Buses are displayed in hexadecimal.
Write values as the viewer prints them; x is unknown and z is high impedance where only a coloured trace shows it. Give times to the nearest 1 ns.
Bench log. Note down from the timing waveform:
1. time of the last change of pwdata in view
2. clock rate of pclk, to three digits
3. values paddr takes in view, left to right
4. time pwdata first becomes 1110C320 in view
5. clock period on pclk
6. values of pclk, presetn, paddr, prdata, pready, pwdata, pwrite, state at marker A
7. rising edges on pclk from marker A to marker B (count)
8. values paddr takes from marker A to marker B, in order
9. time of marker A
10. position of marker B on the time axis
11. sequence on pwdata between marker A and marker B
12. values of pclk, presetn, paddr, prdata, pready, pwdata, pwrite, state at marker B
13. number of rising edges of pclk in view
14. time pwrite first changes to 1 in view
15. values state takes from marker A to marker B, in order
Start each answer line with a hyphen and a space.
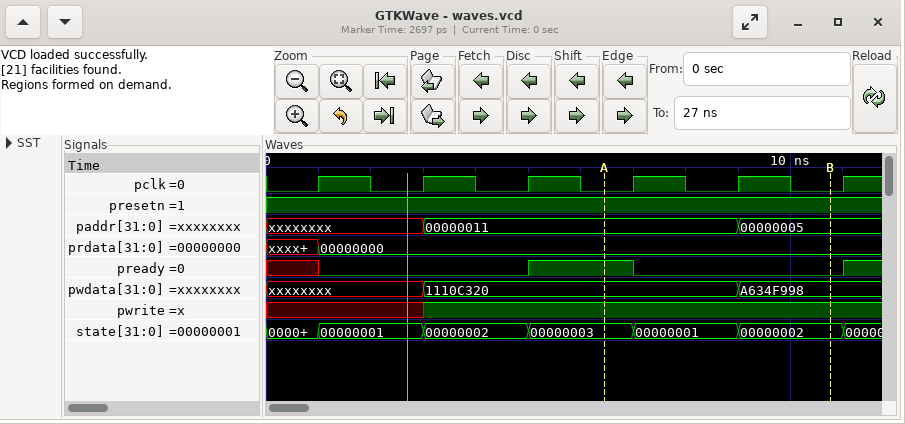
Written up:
- 9 ns
- 500 MHz
- xxxxxxxx, 00000011, 00000005
- 3 ns
- 2 ns
- pclk=0, presetn=1, paddr=00000011, prdata=00000000, pready=1, pwdata=1110C320, pwrite=1, state=00000003
- 2
- 00000011, 00000005
- 6 ns
- 11 ns
- 1110C320, A634F998
- pclk=0, presetn=1, paddr=00000005, prdata=00000000, pready=0, pwdata=A634F998, pwrite=1, state=00000002
- 6
- 3 ns
- 00000003, 00000001, 00000002
